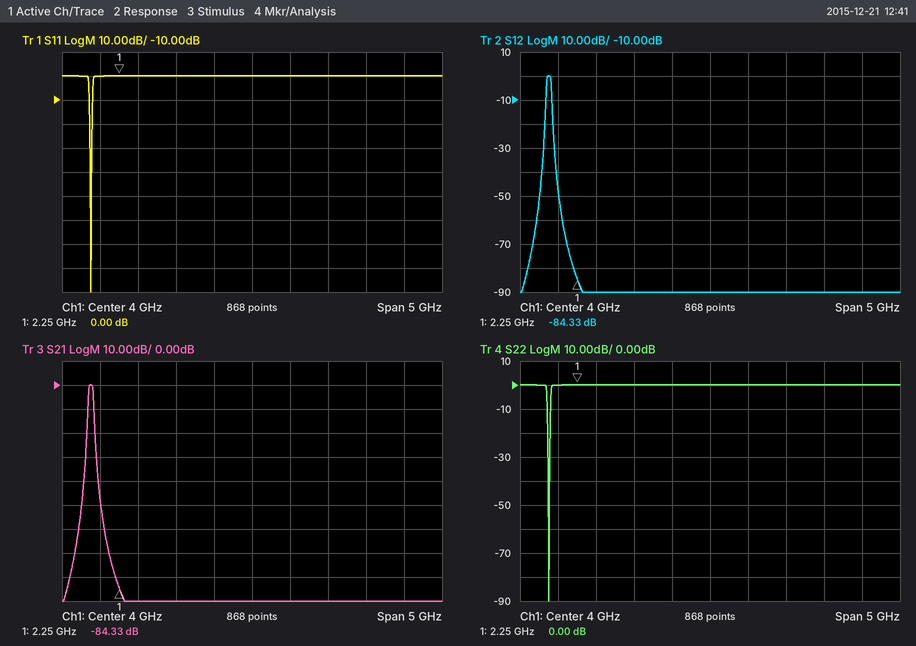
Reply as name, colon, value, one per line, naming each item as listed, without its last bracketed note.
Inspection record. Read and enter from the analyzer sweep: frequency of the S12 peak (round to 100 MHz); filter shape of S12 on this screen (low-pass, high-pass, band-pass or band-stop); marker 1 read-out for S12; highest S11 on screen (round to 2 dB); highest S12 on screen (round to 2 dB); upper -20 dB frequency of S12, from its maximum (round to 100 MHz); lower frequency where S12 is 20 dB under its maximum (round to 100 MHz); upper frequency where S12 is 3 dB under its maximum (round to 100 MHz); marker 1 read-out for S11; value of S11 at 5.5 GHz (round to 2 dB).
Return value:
frequency of the S12 peak: 1.9 GHz
filter shape of S12 on this screen: band-pass
marker 1 read-out for S12: -84.33 dB
highest S11 on screen: 0 dB
highest S12 on screen: 0 dB
upper -20 dB frequency of S12, from its maximum: 1.9 GHz
lower frequency where S12 is 20 dB under its maximum: 1.8 GHz
upper frequency where S12 is 3 dB under its maximum: 1.9 GHz
marker 1 read-out for S11: 0.00 dB
value of S11 at 5.5 GHz: 0 dB
